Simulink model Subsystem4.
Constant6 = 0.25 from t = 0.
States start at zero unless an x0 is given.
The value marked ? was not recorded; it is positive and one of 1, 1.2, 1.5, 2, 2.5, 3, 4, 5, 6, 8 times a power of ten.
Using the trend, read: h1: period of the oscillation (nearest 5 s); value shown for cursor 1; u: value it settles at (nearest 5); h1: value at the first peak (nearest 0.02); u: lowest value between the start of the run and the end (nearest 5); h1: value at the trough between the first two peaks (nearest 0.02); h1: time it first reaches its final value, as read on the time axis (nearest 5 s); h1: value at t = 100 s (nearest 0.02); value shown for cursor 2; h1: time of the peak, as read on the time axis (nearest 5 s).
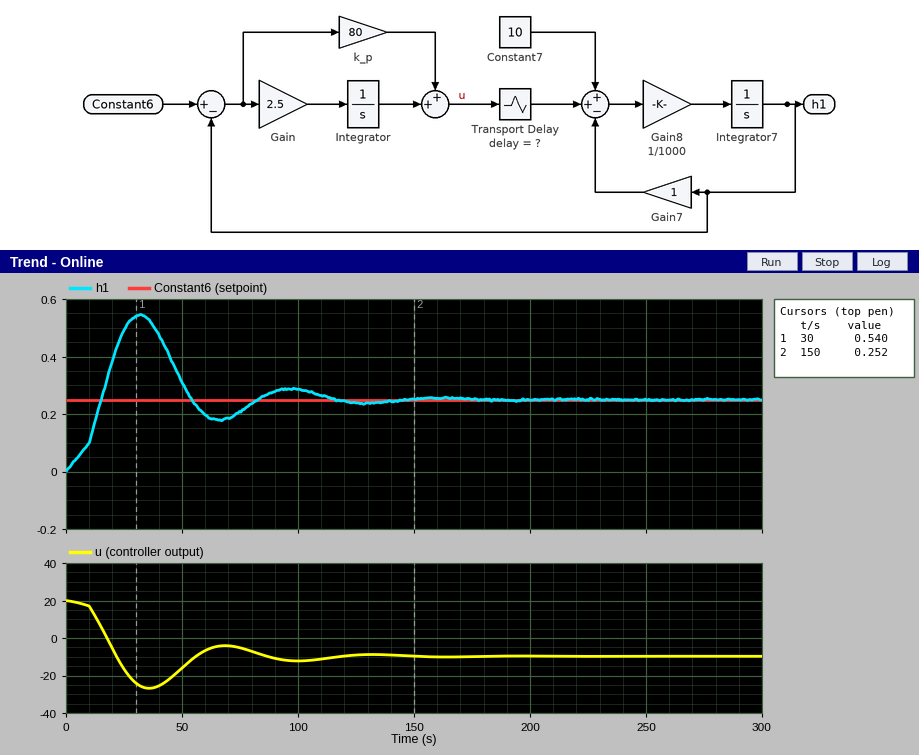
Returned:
65 s
0.540
-10
0.54
-25
0.18
15 s
0.28
0.252
30 s
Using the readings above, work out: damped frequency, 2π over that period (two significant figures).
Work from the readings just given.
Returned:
0.097 rad/s
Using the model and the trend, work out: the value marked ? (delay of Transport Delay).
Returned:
10
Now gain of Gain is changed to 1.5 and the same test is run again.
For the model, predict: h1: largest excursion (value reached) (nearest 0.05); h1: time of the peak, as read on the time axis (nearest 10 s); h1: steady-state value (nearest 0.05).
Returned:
0.50
30 s
0.25
